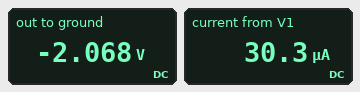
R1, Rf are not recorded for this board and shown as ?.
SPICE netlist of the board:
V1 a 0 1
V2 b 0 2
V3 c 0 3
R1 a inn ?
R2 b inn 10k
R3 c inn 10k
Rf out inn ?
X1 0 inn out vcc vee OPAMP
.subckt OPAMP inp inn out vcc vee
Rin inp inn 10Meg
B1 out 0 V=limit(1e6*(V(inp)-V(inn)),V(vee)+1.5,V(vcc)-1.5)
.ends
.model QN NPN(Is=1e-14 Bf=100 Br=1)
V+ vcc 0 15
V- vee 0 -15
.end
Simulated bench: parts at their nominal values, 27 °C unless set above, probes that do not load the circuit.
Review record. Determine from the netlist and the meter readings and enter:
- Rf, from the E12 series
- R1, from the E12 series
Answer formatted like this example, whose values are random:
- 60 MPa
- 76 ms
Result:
- 3.9 kΩ
- 33 kΩ
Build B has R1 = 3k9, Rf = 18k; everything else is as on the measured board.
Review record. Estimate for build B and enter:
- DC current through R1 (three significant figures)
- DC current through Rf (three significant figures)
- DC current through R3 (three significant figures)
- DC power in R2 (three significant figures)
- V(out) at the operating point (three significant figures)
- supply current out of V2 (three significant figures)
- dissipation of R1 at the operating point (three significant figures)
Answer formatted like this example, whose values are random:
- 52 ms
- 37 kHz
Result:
- 253 µA
- 751 µA
- 299 µA
- 395 µW
- -13.5 V
- 199 µA
- 250 µW
